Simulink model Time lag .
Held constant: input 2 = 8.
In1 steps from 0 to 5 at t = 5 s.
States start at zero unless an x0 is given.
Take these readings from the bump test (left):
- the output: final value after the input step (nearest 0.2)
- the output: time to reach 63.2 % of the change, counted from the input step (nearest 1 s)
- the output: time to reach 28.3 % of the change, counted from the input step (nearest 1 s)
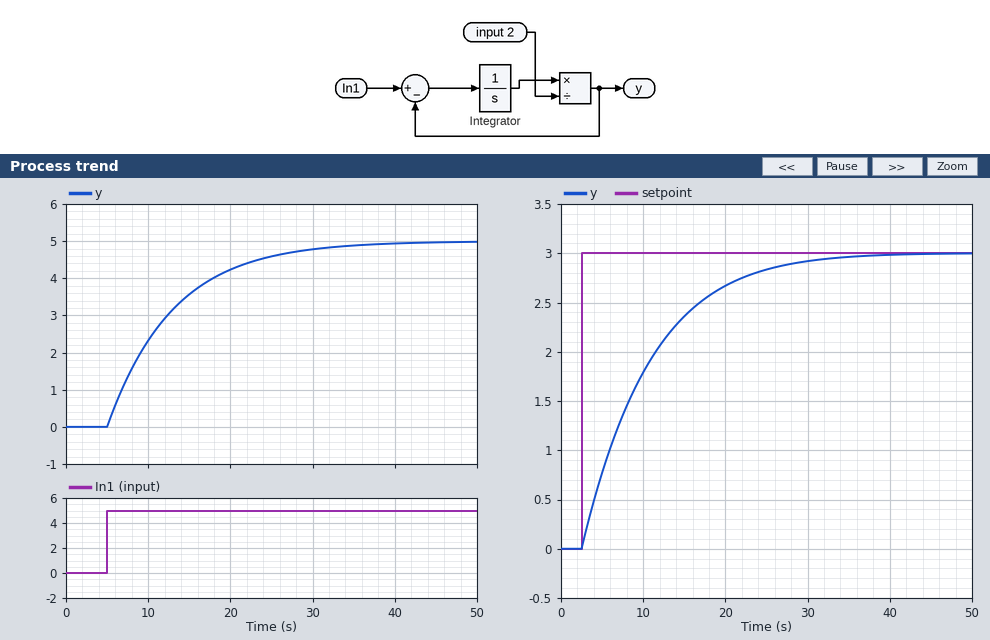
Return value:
5.0
8 s
3 s
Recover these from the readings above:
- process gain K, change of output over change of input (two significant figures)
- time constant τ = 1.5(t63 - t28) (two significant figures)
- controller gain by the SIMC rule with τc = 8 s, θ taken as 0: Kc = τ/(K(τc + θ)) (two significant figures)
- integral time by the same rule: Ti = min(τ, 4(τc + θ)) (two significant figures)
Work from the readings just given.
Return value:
1.0
7.5 s
0.94
7.5 s
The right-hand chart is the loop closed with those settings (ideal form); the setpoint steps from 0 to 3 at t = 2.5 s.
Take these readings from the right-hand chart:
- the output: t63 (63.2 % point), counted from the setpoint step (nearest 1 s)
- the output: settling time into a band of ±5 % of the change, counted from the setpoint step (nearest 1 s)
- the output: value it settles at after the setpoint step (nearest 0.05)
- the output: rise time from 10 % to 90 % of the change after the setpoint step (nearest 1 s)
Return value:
8 s
23 s
3.00
17 s
